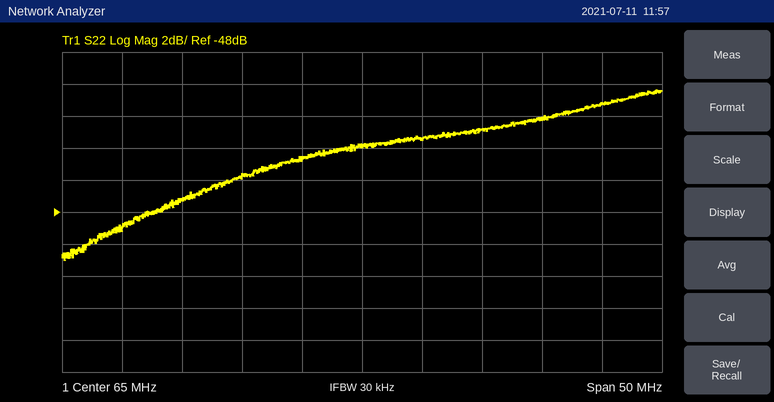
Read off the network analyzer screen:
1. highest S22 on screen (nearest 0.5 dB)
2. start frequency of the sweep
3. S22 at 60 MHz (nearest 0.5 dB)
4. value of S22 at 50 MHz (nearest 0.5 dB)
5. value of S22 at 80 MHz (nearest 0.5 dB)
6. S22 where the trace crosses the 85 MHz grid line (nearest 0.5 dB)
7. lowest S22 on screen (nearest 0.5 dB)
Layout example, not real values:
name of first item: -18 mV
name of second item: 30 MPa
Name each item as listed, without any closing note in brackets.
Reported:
highest S22 on screen: -40.5 dB
start frequency of the sweep: 40 MHz
S22 at 60 MHz: -44.5 dB
value of S22 at 50 MHz: -47.0 dB
value of S22 at 80 MHz: -42.0 dB
S22 where the trace crosses the 85 MHz grid line: -41.0 dB
lowest S22 on screen: -51.0 dB
